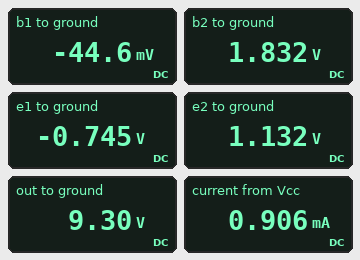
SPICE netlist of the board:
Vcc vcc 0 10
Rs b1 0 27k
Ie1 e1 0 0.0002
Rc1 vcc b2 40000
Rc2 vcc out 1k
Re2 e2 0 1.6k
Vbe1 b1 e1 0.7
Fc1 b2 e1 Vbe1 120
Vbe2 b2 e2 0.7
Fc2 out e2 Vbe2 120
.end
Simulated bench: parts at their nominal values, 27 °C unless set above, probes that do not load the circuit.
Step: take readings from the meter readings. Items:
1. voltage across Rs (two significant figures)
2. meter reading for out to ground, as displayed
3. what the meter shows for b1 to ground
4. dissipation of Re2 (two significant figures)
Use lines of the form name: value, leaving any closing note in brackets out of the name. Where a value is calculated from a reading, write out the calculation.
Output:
voltage across Rs: 0 V - (-44.6 mV) = 45 mV
meter reading for out to ground, as displayed: 9.30 V
what the meter shows for b1 to ground: -44.6 mV
dissipation of Re2: (1.132 V)^2 / 1.6 kΩ = 800 µW
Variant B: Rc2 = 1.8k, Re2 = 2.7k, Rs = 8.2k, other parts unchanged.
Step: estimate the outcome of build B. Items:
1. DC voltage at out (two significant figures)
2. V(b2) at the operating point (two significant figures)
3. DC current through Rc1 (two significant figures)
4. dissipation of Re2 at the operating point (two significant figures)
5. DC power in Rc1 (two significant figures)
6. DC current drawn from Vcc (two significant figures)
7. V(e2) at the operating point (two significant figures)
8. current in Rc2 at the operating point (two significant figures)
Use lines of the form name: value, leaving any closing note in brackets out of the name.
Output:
DC voltage at out: 9.2 V
V(b2) at the operating point: 1.9 V
DC current through Rc1: 200 µA
dissipation of Re2 at the operating point: 550 µW
DC power in Rc1: 1.6 mW
DC current drawn from Vcc: 650 µA
V(e2) at the operating point: 1.2 V
current in Rc2 at the operating point: 450 µA
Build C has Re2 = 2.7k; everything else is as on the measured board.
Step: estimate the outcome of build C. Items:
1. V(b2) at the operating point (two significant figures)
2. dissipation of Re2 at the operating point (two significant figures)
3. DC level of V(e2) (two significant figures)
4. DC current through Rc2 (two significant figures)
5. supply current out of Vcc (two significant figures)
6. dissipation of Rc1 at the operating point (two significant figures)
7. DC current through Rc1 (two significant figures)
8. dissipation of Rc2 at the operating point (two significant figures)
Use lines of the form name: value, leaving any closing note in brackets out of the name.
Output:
V(b2) at the operating point: 1.9 V
dissipation of Re2 at the operating point: 550 µW
DC level of V(e2): 1.2 V
DC current through Rc2: 450 µA
supply current out of Vcc: 650 µA
dissipation of Rc1 at the operating point: 1.6 mW
DC current through Rc1: 200 µA
dissipation of Rc2 at the operating point: 200 µW
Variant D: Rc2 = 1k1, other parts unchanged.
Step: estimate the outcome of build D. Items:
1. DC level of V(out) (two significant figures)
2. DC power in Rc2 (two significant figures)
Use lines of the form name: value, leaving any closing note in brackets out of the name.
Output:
DC level of V(out): 9.2 V
DC power in Rc2: 540 µW
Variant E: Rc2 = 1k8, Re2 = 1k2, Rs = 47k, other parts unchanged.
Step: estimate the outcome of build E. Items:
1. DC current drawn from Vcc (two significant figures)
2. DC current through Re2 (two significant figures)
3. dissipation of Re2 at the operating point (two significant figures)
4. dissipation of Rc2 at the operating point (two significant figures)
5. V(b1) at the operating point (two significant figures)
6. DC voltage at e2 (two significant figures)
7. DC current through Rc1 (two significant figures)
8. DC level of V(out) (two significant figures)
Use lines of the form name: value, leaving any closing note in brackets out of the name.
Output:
DC current drawn from Vcc: 1.1 mA
DC current through Re2: 890 µA
dissipation of Re2 at the operating point: 960 µW
dissipation of Rc2 at the operating point: 1.4 mW
V(b1) at the operating point: -78 mV
DC voltage at e2: 1.1 V
DC current through Rc1: 210 µA
DC level of V(out): 8.4 V
